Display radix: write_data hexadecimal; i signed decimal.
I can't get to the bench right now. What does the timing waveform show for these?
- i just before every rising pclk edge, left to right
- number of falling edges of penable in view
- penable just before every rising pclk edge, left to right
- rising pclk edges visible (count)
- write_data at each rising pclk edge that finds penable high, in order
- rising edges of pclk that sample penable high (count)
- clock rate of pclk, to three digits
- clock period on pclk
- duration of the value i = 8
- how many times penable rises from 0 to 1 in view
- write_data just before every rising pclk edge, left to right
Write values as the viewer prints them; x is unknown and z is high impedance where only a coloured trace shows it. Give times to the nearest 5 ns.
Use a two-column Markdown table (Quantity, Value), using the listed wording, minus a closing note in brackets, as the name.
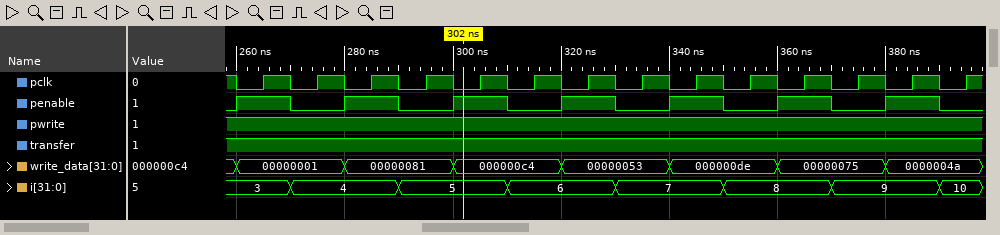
| Quantity | Value |
|---|---|
| i just before every rising pclk edge, left to right | 3, 4, 4, 5, 5, 6, 6, 7, 7, 8, 8, 9, 9, 10 |
| number of falling edges of penable in view | 7 |
| penable just before every rising pclk edge, left to right | 1 0 1 0 1 0 1 0 1 0 1 0 1 0 |
| rising pclk edges visible | 14 |
| write_data at each rising pclk edge that finds penable high, in order | 00000001, 00000081, 000000c4, 00000053, 000000de, 00000075, 0000004a |
| rising edges of pclk that sample penable high | 7 |
| clock rate of pclk, to three digits | 100 MHz |
| clock period on pclk | 10 ns |
| duration of the value i = 8 | 20 ns |
| how many times penable rises from 0 to 1 in view | 7 |
| write_data just before every rising pclk edge, left to right | 00000001, 00000001, 00000081, 00000081, 000000c4, 000000c4, 00000053, 00000053, 000000de, 000000de, 00000075, 00000075, 0000004a, 0000004a |
